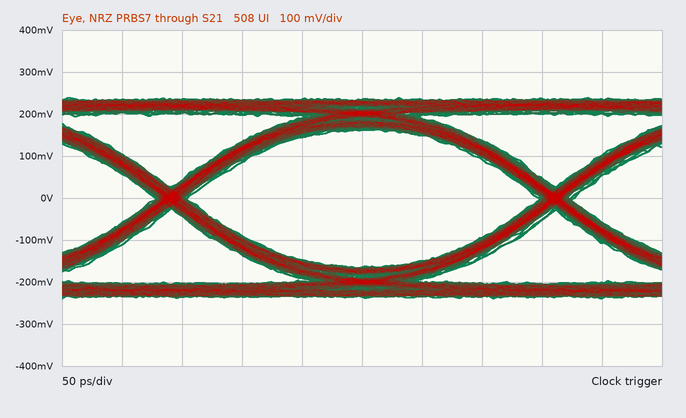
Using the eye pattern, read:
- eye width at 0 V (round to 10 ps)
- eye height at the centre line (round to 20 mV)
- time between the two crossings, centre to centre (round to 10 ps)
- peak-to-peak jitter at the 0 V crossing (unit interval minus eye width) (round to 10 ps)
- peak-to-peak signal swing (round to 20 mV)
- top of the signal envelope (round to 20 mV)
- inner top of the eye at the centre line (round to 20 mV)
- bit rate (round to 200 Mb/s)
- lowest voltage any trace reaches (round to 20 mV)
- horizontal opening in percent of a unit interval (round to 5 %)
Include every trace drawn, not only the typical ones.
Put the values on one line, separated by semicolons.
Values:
290 ps; 320 mV; 320 ps; 30 ps; 480 mV; 240 mV; 160 mV; 3.2 Gb/s; -240 mV; 90 %
